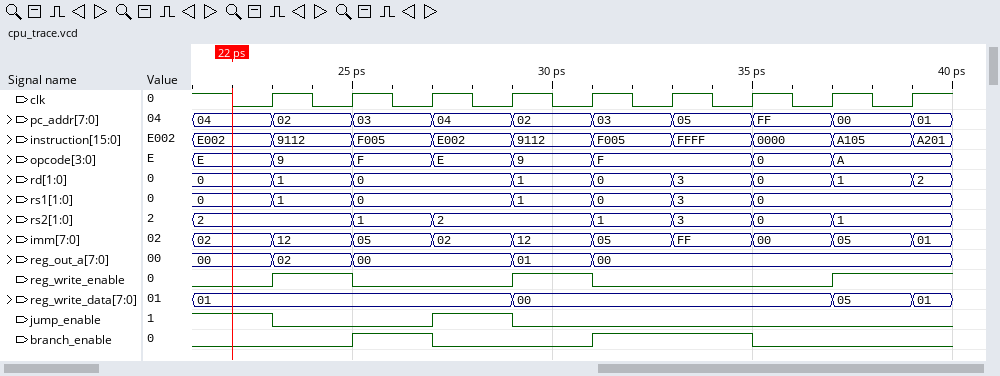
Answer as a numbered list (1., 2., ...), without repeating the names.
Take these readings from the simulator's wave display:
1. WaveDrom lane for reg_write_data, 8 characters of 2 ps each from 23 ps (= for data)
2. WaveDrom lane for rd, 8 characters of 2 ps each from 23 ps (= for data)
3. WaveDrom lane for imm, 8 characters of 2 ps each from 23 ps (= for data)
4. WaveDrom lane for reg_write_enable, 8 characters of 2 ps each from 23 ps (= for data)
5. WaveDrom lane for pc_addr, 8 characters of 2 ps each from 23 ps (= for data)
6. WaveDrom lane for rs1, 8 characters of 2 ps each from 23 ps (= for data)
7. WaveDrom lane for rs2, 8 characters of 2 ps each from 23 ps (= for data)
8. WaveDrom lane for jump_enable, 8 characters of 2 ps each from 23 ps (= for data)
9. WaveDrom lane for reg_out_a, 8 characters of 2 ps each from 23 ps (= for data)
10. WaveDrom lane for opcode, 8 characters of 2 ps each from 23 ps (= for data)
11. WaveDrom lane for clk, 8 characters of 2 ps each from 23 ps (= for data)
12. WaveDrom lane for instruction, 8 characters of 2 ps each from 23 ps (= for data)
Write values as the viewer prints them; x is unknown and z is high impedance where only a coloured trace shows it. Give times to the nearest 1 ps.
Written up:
1. {name: 'reg_write_data', wave: '=..=...=', data: '01 00 05'}
2. {name: 'rd', wave: '==.=====', data: '1 0 1 0 3 0 1'}
3. {name: 'imm', wave: '========', data: '12 05 02 12 05 FF 00 05'}
4. {name: 'reg_write_enable', wave: '10.10..1'}
5. {name: 'pc_addr', wave: '========', data: '02 03 04 02 03 05 FF 00'}
6. {name: 'rs1', wave: '==.====.', data: '1 0 1 0 3 0'}
7. {name: 'rs2', wave: '===.====', data: '2 1 2 1 3 0 1'}
8. {name: 'jump_enable', wave: '0.10....'}
9. {name: 'reg_out_a', wave: '==.==...', data: '02 00 01 00'}
10. {name: 'opcode', wave: '=====.==', data: '9 F E 9 F 0 A'}
11. {name: 'clk', wave: 'p.......'}
12. {name: 'instruction', wave: '========', data: '9112 F005 E002 9112 F005 FFFF 0000 A105'}
